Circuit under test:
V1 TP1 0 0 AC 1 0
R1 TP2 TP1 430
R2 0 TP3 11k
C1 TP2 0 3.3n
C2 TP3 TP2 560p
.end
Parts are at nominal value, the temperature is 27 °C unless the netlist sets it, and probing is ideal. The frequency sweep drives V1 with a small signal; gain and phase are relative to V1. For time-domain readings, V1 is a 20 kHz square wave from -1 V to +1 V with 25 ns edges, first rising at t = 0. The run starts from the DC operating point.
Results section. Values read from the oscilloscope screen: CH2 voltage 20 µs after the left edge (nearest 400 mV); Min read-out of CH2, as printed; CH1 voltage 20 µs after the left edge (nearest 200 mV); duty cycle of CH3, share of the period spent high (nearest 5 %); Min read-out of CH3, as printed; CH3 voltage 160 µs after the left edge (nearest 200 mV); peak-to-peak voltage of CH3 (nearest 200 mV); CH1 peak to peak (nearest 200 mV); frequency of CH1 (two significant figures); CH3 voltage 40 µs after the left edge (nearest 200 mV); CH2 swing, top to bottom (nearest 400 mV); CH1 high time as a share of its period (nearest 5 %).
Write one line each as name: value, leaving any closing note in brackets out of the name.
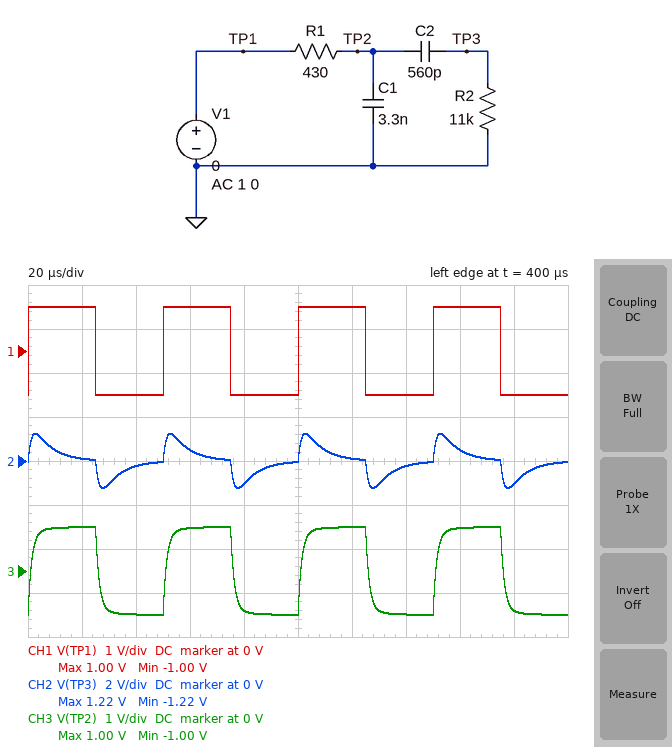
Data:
CH2 voltage 20 µs after the left edge: 0 V
Min read-out of CH2, as printed: -1.22 V
CH1 voltage 20 µs after the left edge: 1.0 V
duty cycle of CH3, share of the period spent high: 50 %
Min read-out of CH3, as printed: -1.00 V
CH3 voltage 160 µs after the left edge: 1.0 V
peak-to-peak voltage of CH3: 2.0 V
CH1 peak to peak: 2.0 V
frequency of CH1: 20 kHz
CH3 voltage 40 µs after the left edge: -1.0 V
CH2 swing, top to bottom: 2.4 V
CH1 high time as a share of its period: 50 %
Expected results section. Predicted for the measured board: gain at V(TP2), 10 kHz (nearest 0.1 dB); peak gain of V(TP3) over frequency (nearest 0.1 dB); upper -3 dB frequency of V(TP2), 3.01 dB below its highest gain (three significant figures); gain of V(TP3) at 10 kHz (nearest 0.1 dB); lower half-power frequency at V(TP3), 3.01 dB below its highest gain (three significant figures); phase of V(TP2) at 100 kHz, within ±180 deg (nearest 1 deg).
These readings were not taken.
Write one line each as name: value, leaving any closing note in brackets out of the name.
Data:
gain at V(TP2), 10 kHz: -0.1 dB
peak gain of V(TP3) over frequency: -2.1 dB
upper -3 dB frequency of V(TP2), 3.01 dB below its highest gain: 107 kHz
gain of V(TP3) at 10 kHz: -8.9 dB
lower half-power frequency at V(TP3), 3.01 dB below its highest gain: 18.1 kHz
phase of V(TP2) at 100 kHz, within ±180 deg: -41 deg
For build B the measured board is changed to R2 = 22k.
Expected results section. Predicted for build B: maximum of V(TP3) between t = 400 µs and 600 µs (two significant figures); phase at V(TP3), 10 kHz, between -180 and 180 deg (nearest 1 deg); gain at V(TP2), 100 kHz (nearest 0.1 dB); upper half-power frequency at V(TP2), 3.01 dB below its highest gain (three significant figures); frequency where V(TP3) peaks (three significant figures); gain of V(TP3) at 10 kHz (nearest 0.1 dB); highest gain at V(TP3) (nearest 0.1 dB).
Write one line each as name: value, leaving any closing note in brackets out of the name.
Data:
maximum of V(TP3) between t = 400 µs and 600 µs: 1.3 V
phase at V(TP3), 10 kHz, between -180 and 180 deg: 47 deg
gain at V(TP2), 100 kHz: -2.6 dB
upper half-power frequency at V(TP2), 3.01 dB below its highest gain: 110 kHz
frequency where V(TP3) peaks: 38.1 kHz
gain of V(TP3) at 10 kHz: -4.4 dB
highest gain at V(TP3): -1.1 dB
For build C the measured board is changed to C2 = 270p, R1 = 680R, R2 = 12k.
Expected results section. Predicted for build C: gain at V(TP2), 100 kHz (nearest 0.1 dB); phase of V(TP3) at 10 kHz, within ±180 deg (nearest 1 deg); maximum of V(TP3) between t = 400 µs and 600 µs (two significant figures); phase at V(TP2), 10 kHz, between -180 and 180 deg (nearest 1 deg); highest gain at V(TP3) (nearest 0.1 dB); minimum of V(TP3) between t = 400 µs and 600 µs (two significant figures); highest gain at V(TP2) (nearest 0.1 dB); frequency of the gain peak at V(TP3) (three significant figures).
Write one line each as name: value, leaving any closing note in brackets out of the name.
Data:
gain at V(TP2), 100 kHz: -5.0 dB
phase of V(TP3) at 10 kHz, within ±180 deg: 70 deg
maximum of V(TP3) between t = 400 µs and 600 µs: 850 mV
phase at V(TP2), 10 kHz, between -180 and 180 deg: -9 deg
highest gain at V(TP3): -4.9 dB
minimum of V(TP3) between t = 400 µs and 600 µs: -850 mV
highest gain at V(TP2): 0 dB
frequency of the gain peak at V(TP3): 59.0 kHz
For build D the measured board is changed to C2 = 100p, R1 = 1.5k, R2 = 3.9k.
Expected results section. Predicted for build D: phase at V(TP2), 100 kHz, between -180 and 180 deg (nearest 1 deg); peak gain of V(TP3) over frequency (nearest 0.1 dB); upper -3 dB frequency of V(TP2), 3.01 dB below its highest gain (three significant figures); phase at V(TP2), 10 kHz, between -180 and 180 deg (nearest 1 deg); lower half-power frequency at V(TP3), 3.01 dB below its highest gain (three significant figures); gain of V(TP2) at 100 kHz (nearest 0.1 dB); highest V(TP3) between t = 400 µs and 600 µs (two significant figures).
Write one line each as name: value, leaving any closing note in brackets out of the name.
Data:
phase at V(TP2), 100 kHz, between -180 and 180 deg: -72 deg
peak gain of V(TP3) over frequency: -23.0 dB
upper -3 dB frequency of V(TP2), 3.01 dB below its highest gain: 31.1 kHz
phase at V(TP2), 10 kHz, between -180 and 180 deg: -18 deg
lower half-power frequency at V(TP3), 3.01 dB below its highest gain: 27.3 kHz
gain of V(TP2) at 100 kHz: -10.5 dB
highest V(TP3) between t = 400 µs and 600 µs: 120 mV
